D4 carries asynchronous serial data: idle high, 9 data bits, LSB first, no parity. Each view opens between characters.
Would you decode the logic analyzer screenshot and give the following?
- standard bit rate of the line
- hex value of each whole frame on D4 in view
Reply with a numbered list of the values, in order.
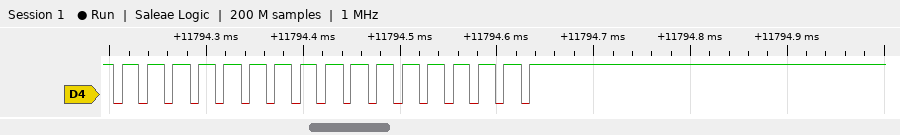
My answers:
1. 115200 baud
2. DB, DB, DB, DB, 1FF
